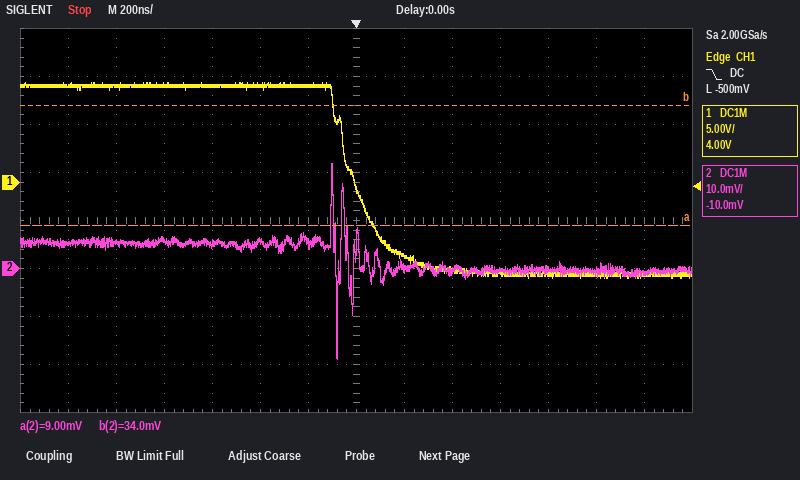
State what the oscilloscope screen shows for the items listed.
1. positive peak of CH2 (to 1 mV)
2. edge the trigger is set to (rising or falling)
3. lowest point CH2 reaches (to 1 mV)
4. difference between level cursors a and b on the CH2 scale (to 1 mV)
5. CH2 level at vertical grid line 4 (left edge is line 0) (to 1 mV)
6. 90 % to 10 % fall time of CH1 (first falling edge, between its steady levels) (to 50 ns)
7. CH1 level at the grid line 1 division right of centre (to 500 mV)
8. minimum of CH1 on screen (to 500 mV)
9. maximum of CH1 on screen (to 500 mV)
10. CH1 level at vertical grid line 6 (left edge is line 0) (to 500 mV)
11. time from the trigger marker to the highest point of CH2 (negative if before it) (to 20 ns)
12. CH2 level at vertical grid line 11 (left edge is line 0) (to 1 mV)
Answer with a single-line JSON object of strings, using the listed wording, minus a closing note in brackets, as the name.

{"positive peak of CH2": "22 mV", "edge the trigger is set to": "falling", "lowest point CH2 reaches": "-19 mV", "difference between level cursors a and b on the CH2 scale": "25 mV", "CH2 level at vertical grid line 4 (left edge is line 0)": "5 mV", "90 % to 10 % fall time of CH1 (first falling edge, between its steady levels)": "300 ns", "CH1 level at the grid line 1 division right of centre": "-7.5 V", "minimum of CH1 on screen": "-10.0 V", "maximum of CH1 on screen": "10.5 V", "CH1 level at vertical grid line 6 (left edge is line 0)": "10.0 V", "time from the trigger marker to the highest point of CH2 (negative if before it)": "-100 ns", "CH2 level at vertical grid line 11 (left edge is line 0)": "0 mV"}
